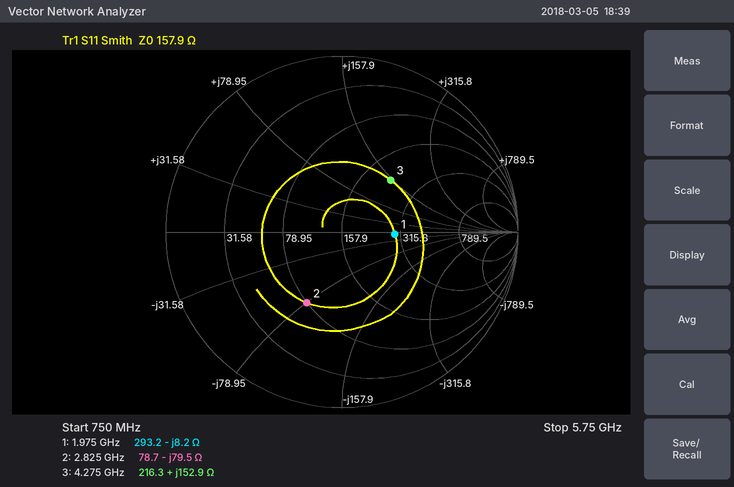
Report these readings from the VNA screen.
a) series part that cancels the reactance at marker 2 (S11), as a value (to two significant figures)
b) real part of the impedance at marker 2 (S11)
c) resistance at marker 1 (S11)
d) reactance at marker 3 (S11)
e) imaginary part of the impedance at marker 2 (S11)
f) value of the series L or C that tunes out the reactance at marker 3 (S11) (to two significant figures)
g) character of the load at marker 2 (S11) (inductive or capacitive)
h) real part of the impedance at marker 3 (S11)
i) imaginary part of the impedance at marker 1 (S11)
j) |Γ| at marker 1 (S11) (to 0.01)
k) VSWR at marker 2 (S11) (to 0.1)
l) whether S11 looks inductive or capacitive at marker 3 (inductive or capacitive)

4.5 nH
78.7 Ω
293.2 Ω
+152.9 Ω
-79.5 Ω
240 fF
capacitive
216.3 Ω
-8.2 Ω
0.30
2.6
inductive
